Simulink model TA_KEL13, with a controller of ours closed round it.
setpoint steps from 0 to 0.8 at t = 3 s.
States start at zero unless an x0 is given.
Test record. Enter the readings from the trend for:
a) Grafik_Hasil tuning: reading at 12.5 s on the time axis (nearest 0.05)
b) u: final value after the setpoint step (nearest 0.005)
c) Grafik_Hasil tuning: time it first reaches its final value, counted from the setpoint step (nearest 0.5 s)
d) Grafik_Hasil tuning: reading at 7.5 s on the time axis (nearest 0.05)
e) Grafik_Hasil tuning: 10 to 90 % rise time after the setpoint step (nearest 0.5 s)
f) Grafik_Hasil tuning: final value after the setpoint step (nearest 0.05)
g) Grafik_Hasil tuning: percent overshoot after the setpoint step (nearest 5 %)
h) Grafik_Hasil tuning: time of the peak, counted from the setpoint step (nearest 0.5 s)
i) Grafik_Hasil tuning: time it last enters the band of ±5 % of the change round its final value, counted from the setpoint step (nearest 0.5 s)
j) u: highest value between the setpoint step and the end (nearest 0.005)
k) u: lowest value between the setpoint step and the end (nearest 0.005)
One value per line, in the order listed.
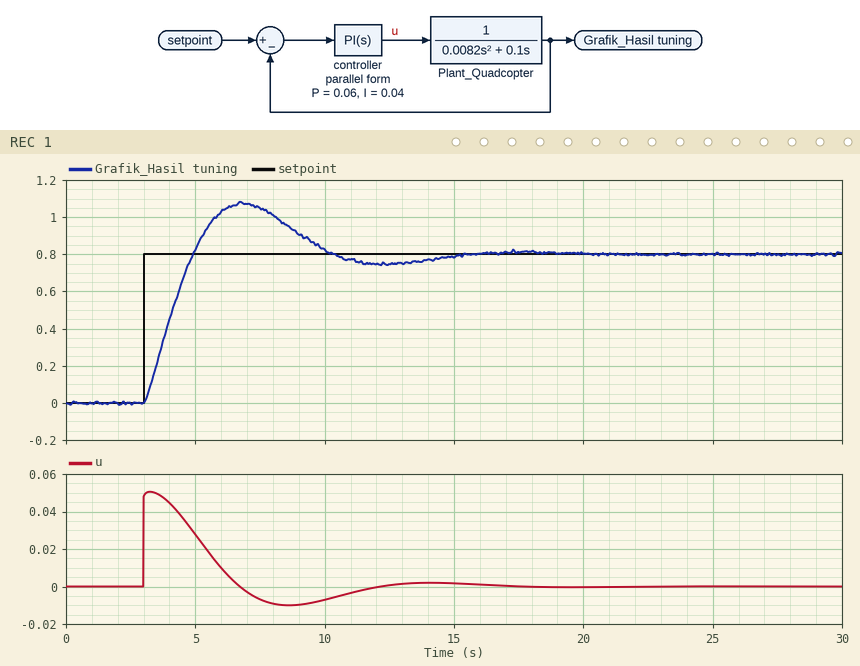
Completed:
0.75
0.000
2.0 s
1.05
1.5 s
0.80
35 %
4.0 s
10.5 s
0.050
-0.010
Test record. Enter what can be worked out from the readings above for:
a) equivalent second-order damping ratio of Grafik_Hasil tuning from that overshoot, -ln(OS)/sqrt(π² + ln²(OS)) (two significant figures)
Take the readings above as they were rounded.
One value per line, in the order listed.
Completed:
0.32
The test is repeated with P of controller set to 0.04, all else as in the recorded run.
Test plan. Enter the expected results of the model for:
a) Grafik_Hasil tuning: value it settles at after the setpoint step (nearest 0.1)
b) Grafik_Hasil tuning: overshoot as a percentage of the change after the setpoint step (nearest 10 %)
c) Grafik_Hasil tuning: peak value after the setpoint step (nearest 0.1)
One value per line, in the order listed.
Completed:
0.8
50 %
1.2
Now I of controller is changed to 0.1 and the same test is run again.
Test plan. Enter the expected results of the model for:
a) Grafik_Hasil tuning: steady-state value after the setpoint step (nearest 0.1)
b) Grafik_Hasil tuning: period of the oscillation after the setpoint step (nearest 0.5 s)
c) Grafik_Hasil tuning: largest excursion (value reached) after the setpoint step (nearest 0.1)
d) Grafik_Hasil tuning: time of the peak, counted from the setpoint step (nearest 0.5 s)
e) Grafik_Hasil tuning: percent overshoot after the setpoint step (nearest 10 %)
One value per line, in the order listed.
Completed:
0.8
6.5 s
1.2
2.5 s
50 %
